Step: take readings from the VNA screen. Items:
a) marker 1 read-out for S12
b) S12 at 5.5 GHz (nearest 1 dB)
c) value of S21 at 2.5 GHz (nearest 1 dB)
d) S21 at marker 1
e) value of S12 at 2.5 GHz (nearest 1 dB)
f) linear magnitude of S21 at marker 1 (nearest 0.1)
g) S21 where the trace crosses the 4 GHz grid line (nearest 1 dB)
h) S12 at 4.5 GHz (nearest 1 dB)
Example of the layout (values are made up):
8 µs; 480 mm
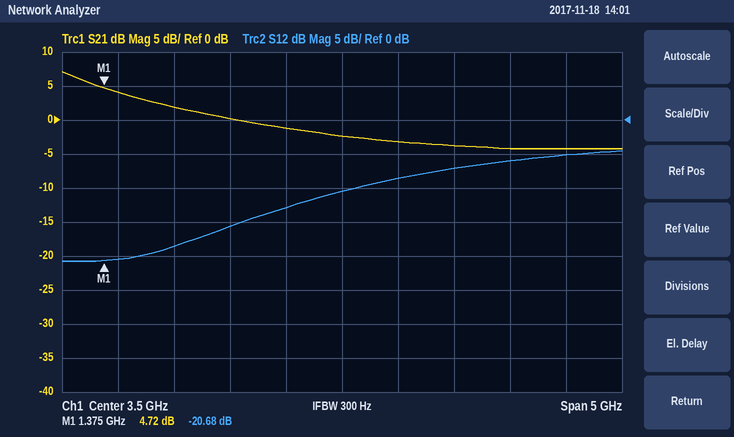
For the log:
-20.68 dB; -5 dB; 0 dB; 4.72 dB; -16 dB; 1.7; -3 dB; -7 dB
